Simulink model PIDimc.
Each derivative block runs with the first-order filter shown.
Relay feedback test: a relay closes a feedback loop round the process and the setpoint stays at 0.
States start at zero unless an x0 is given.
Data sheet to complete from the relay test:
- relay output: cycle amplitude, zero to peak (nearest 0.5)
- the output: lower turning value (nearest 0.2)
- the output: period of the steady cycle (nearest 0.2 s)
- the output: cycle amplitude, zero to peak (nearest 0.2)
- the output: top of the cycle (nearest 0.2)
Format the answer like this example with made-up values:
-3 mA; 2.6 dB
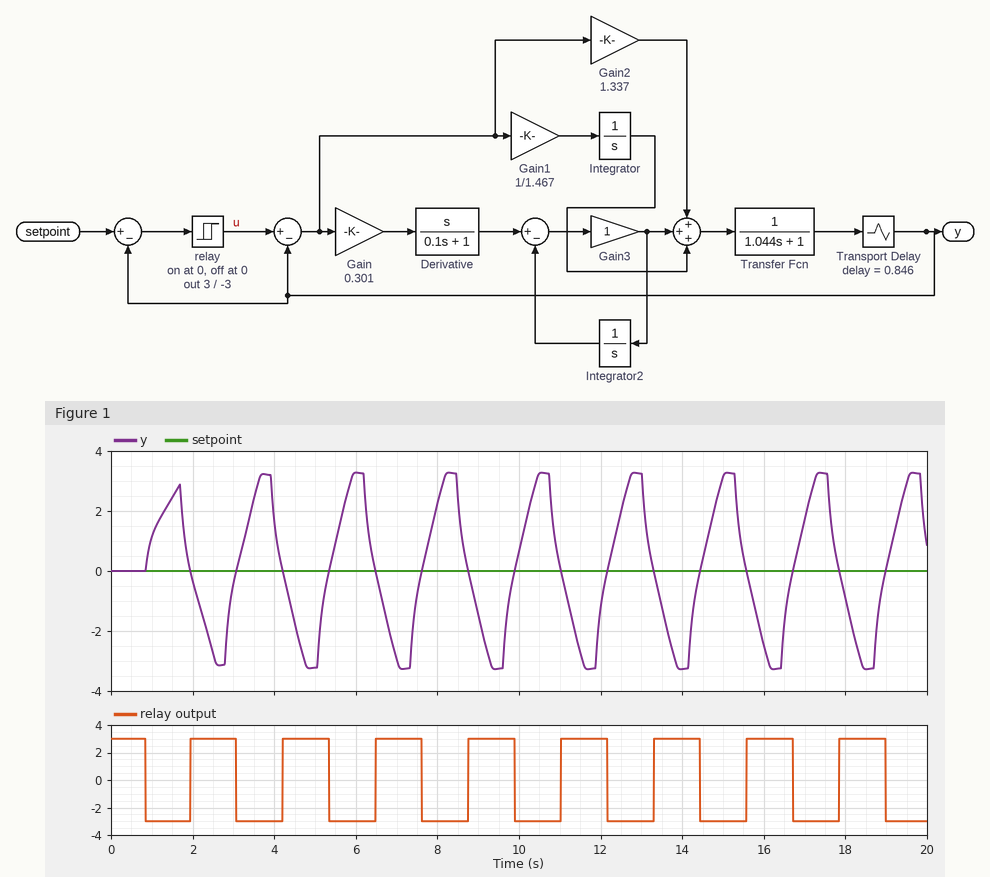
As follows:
3.0; -3.2; 2.2 s; 3.2; 3.2
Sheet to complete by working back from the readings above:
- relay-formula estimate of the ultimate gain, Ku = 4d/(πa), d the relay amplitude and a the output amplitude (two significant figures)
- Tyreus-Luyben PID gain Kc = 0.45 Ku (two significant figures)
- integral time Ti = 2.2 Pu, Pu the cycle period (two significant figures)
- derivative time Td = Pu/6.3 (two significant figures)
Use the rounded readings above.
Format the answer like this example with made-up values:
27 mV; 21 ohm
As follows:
1.2; 0.54; 4.8 s; 0.35 s
